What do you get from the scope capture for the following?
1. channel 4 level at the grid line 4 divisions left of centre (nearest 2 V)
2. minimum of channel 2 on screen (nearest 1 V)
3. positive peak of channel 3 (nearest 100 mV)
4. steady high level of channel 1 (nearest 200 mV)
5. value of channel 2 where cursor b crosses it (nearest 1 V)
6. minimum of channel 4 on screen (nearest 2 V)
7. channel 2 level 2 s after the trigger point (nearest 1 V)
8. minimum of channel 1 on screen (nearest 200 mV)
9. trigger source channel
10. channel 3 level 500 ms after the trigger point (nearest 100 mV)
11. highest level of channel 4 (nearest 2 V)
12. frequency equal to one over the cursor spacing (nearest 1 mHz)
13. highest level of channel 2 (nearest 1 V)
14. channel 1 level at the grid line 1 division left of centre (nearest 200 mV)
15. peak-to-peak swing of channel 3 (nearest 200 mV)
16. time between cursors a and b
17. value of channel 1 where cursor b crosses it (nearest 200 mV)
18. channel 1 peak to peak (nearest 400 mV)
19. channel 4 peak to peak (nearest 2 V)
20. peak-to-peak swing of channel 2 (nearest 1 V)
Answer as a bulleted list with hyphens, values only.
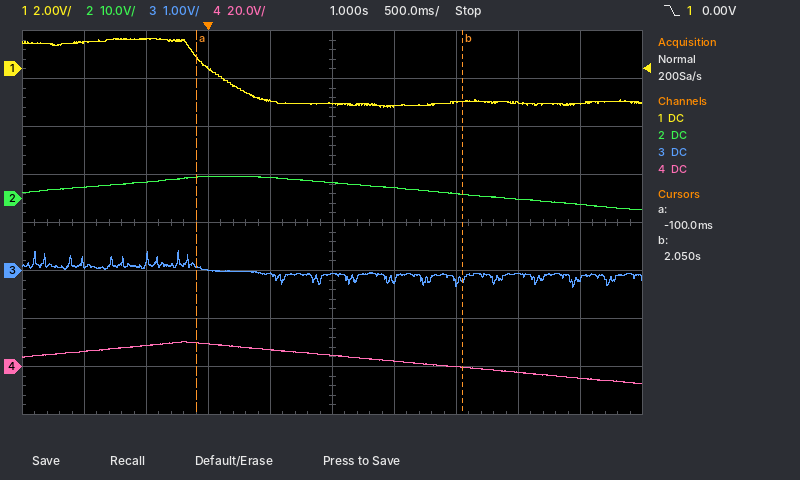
- 6 V
- -2 V
- 400 mV
- 1.2 V
- 1 V
- -8 V
- 1 V
- -1.6 V
- channel 1
- -100 mV
- 10 V
- 465 mHz
- 5 V
- -1.4 V
- 800 mV
- 2.15 s
- -1.4 V
- 2.8 V
- 18 V
- 7 V
